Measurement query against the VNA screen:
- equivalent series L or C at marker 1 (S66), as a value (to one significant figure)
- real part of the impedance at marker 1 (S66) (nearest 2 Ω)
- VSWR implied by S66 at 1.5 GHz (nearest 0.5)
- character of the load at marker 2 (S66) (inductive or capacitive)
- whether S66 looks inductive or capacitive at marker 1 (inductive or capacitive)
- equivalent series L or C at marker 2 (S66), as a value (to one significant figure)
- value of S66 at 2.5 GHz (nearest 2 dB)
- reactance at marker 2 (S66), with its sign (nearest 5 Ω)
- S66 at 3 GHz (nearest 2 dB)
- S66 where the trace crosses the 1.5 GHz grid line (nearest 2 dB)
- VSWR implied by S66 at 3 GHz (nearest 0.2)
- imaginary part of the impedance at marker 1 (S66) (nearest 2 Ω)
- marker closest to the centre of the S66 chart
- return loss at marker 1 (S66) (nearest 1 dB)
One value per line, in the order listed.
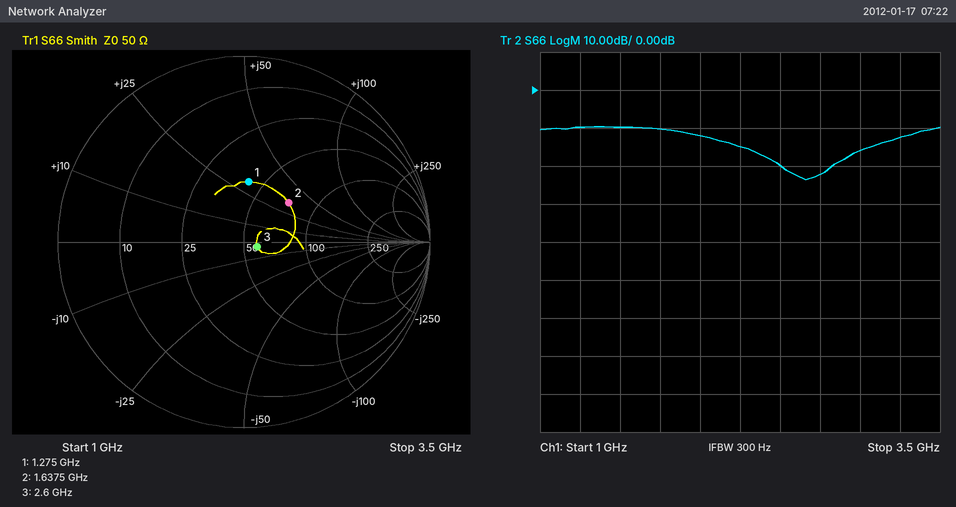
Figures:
4 nH
42 Ω
2.0
inductive
inductive
3 nH
-20 dB
+35 Ω
-16 dB
-10 dB
1.4
+30 Ω
marker 3
10 dB
